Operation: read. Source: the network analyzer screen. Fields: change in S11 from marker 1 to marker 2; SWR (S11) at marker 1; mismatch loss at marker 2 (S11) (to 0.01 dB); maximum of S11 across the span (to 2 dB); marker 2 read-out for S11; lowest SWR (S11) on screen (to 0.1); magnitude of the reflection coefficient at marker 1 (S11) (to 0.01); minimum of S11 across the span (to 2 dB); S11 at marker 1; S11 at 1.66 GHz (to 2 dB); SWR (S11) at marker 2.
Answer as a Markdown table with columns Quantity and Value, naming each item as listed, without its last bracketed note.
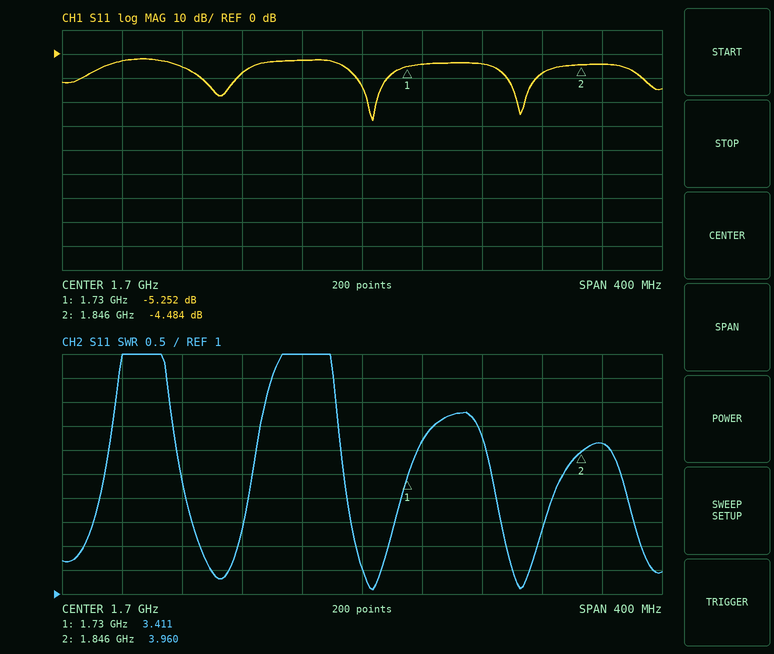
| Quantity | Value |
|---|---|
| change in S11 from marker 1 to marker 2 | 0.768 dB |
| SWR (S11) at marker 1 | 3.411 |
| mismatch loss at marker 2 (S11) | 1.91 dB |
| maximum of S11 across the span | -2 dB |
| marker 2 read-out for S11 | -4.484 dB |
| lowest SWR (S11) on screen | 1.1 |
| magnitude of the reflection coefficient at marker 1 (S11) | 0.55 |
| minimum of S11 across the span | -28 dB |
| S11 at marker 1 | -5.252 dB |
| S11 at 1.66 GHz | -2 dB |
| SWR (S11) at marker 2 | 3.960 |
